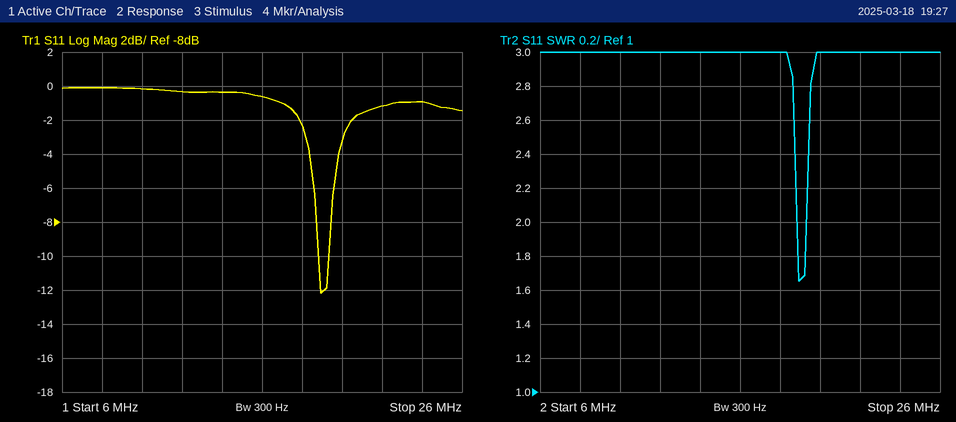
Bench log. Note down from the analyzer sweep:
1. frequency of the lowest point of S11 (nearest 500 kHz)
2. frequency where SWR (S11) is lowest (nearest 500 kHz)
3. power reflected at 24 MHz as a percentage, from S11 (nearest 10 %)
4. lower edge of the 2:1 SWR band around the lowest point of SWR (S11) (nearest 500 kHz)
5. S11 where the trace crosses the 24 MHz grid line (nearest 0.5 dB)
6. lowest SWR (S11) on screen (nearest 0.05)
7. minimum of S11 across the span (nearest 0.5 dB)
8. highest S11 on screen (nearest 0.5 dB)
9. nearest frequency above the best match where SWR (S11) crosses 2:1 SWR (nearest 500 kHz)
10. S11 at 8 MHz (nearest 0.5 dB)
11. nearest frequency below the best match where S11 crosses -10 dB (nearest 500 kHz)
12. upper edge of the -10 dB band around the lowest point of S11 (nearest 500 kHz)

19.0 MHz
19.0 MHz
80 %
19.0 MHz
-1.0 dB
1.65
-12.0 dB
0.0 dB
19.5 MHz
0.0 dB
19.0 MHz
19.5 MHz
